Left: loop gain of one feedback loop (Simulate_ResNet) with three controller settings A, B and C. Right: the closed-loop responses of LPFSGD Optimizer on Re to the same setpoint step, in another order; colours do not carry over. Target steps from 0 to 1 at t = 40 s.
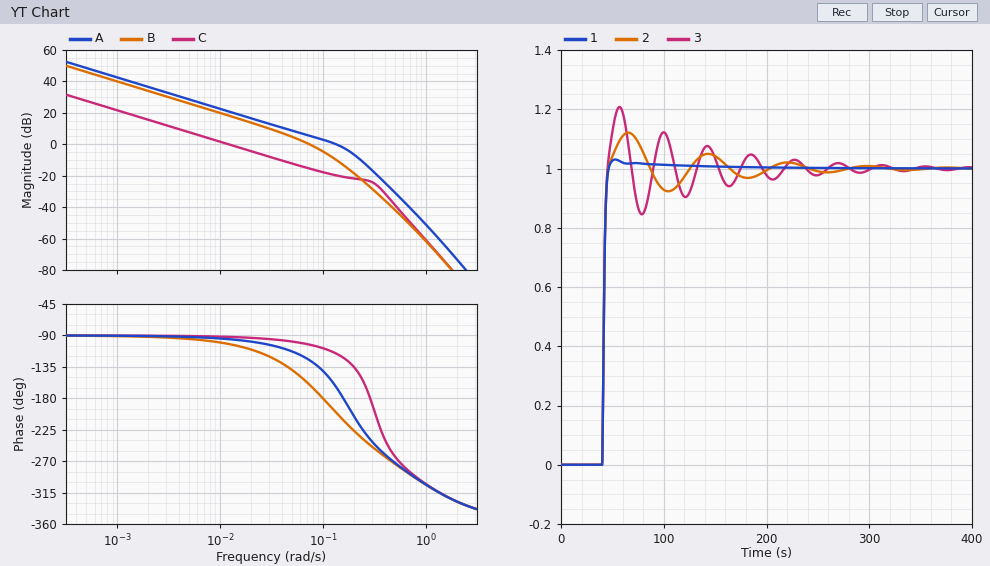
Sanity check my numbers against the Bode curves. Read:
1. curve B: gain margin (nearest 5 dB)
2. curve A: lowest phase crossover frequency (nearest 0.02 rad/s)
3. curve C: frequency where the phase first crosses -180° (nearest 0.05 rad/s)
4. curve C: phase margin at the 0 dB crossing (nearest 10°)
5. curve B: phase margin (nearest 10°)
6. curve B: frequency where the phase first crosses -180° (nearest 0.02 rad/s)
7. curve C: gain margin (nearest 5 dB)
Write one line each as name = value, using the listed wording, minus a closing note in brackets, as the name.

curve B: gain margin = 5 dB
curve A: lowest phase crossover frequency = 0.16 rad/s
curve C: frequency where the phase first crosses -180° = 0.30 rad/s
curve C: phase margin at the 0 dB crossing = 90°
curve B: phase margin = 20°
curve B: frequency where the phase first crosses -180° = 0.10 rad/s
curve C: gain margin = 25 dB
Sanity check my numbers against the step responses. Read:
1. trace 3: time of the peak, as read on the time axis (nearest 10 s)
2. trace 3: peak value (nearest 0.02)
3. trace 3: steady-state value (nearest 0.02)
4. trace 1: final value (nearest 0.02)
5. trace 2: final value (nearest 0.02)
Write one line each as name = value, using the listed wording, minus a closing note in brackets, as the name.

trace 3: time of the peak, as read on the time axis = 60 s
trace 3: peak value = 1.20
trace 3: steady-state value = 1.00
trace 1: final value = 1.00
trace 2: final value = 1.00
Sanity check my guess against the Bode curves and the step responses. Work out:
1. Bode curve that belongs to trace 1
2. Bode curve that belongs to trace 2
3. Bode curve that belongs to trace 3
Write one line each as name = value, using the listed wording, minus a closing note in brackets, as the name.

Bode curve that belongs to trace 1 = C
Bode curve that belongs to trace 2 = B
Bode curve that belongs to trace 3 = A
